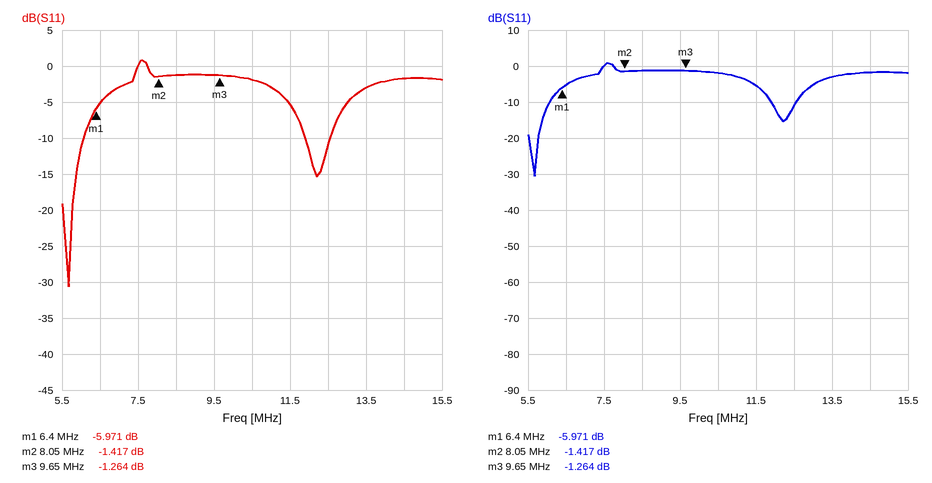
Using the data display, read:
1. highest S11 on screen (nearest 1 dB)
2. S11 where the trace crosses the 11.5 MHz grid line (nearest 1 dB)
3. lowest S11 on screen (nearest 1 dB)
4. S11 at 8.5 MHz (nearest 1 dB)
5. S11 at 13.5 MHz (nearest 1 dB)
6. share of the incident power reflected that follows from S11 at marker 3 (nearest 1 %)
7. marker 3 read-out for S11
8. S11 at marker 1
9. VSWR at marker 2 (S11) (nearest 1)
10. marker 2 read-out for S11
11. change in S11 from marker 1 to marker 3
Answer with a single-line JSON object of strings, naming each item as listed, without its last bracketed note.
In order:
{"highest S11 on screen": "1 dB", "S11 where the trace crosses the 11.5 MHz grid line": "-5 dB", "lowest S11 on screen": "-31 dB", "S11 at 8.5 MHz": "-1 dB", "S11 at 13.5 MHz": "-3 dB", "share of the incident power reflected that follows from S11 at marker 3": "75 %", "marker 3 read-out for S11": "-1.264 dB", "S11 at marker 1": "-5.971 dB", "VSWR at marker 2 (S11)": "12", "marker 2 read-out for S11": "-1.417 dB", "change in S11 from marker 1 to marker 3": "4.707 dB"}
